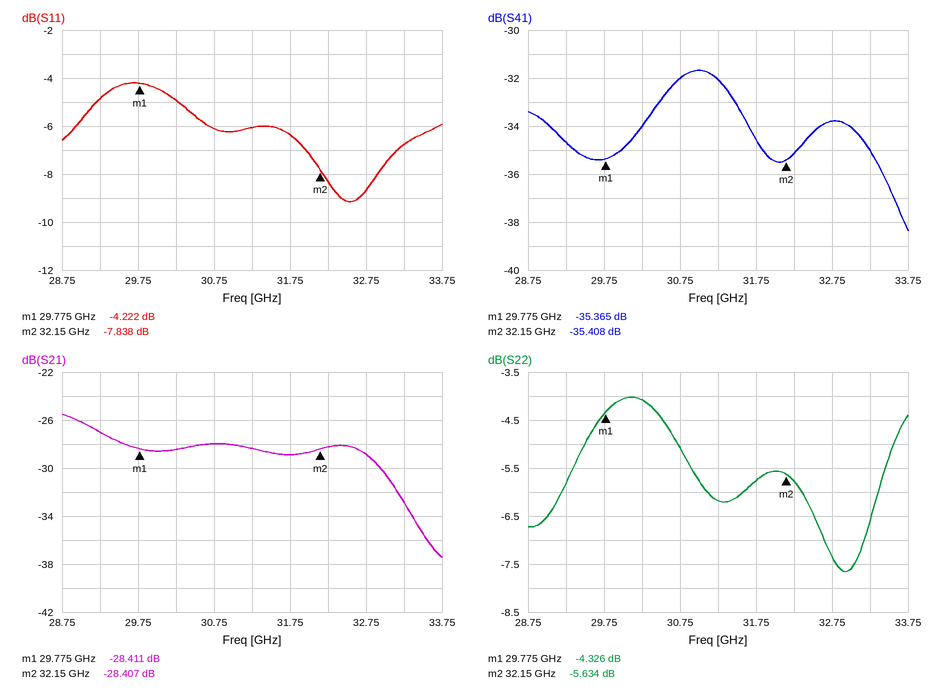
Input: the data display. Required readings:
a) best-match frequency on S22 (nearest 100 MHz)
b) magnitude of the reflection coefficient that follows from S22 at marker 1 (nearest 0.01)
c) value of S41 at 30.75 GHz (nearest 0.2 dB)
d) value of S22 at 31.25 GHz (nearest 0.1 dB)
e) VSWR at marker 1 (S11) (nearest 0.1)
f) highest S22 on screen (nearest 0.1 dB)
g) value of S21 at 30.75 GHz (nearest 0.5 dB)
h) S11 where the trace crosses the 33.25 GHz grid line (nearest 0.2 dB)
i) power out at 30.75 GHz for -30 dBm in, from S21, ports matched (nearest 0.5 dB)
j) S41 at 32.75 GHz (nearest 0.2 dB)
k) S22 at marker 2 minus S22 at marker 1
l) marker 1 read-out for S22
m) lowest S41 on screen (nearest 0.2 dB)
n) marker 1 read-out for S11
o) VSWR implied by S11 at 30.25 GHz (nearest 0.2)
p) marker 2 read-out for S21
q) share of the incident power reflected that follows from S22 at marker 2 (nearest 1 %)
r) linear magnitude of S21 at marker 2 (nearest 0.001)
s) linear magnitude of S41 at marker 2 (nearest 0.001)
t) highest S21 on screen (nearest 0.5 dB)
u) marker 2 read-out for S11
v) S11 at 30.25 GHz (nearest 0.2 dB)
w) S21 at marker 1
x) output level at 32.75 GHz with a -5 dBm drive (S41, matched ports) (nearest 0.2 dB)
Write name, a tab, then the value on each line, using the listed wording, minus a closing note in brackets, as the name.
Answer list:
best-match frequency on S22	32.9 GHz
magnitude of the reflection coefficient that follows from S22 at marker 1	0.61
value of S41 at 30.75 GHz	-32.0 dB
value of S22 at 31.25 GHz	-6.2 dB
VSWR at marker 1 (S11)	4.2
highest S22 on screen	-4.0 dB
value of S21 at 30.75 GHz	-28.0 dB
S11 where the trace crosses the 33.25 GHz grid line	-6.8 dB
power out at 30.75 GHz for -30 dBm in, from S21, ports matched	-58.0 dBm
S41 at 32.75 GHz	-33.8 dB
S22 at marker 2 minus S22 at marker 1	-1.308 dB
marker 1 read-out for S22	-4.326 dB
lowest S41 on screen	-38.4 dB
marker 1 read-out for S11	-4.222 dB
VSWR implied by S11 at 30.25 GHz	3.6
marker 2 read-out for S21	-28.407 dB
share of the incident power reflected that follows from S22 at marker 2	27 %
linear magnitude of S21 at marker 2	0.038
linear magnitude of S41 at marker 2	0.017
highest S21 on screen	-25.5 dB
marker 2 read-out for S11	-7.838 dB
S11 at 30.25 GHz	-5.0 dB
S21 at marker 1	-28.411 dB
output level at 32.75 GHz with a -5 dBm drive (S41, matched ports)	-38.8 dBm
